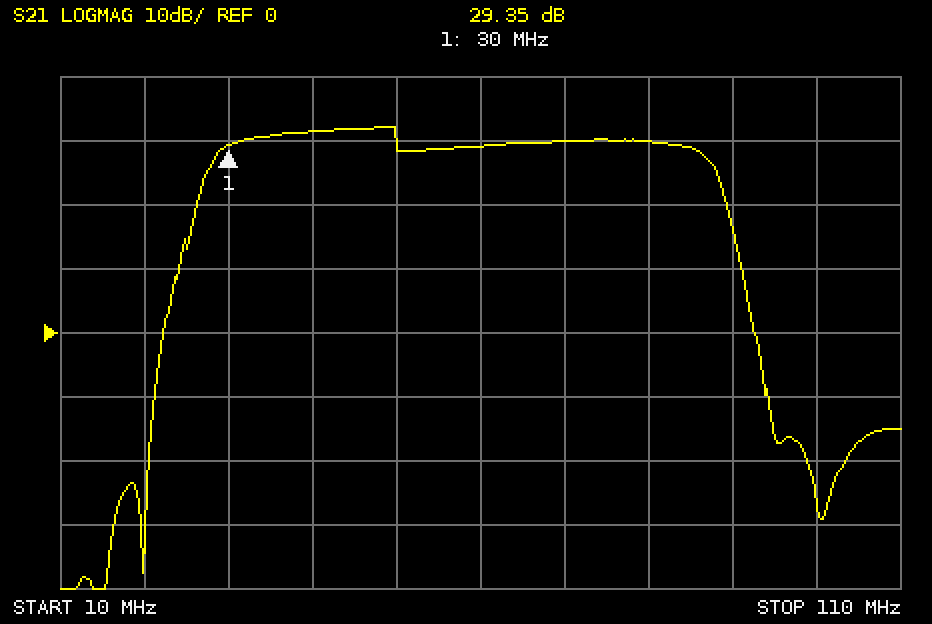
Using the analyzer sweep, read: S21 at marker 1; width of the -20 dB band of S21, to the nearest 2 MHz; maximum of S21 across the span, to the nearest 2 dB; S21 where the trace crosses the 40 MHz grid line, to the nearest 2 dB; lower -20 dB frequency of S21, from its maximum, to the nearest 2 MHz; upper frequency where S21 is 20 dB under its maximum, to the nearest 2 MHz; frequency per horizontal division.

29.35 dB
66 MHz
32 dB
32 dB
24 MHz
90 MHz
10 MHz
